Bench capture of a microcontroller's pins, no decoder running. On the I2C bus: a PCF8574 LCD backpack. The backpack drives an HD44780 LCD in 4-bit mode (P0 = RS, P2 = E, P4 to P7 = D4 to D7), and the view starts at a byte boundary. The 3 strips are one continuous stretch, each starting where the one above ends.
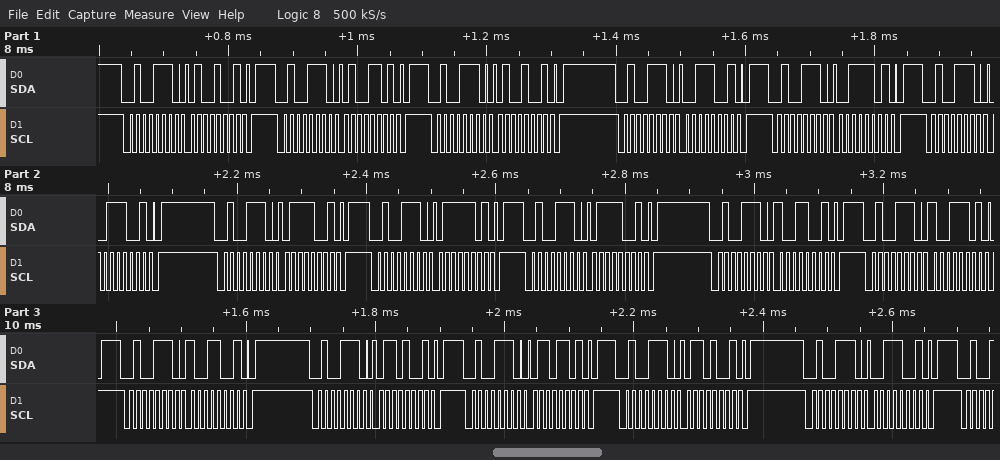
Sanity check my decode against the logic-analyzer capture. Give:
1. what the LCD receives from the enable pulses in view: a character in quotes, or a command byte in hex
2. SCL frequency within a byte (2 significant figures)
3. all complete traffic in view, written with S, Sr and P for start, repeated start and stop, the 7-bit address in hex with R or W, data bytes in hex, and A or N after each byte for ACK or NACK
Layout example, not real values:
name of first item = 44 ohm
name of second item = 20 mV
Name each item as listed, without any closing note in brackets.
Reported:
what the LCD receives from the enable pulses in view: a character in quotes, or a command byte in hex = 'C' 'y'
SCL frequency within a byte = 100 kHz
all complete traffic in view, written with S, Sr and P for start, repeated start and stop, the 7-bit address in hex with R or W, data bytes in hex, and A or N after each byte for ACK or NACK = S 27W A 49 A P S 27W A 4D A P S 27W A 49 A P S 27W A 39 A P S 27W A 3D A P S 27W A 39 A P S 27W A 79 A P S 27W A 7D A P S 27W A 79 A P S 27W A 99 A P S 27W A 9D A P S 27W A 99 A P S 27W A 69 A P S 27W A 6D A P S 27W A 69 A P S 27W A 39 A P
